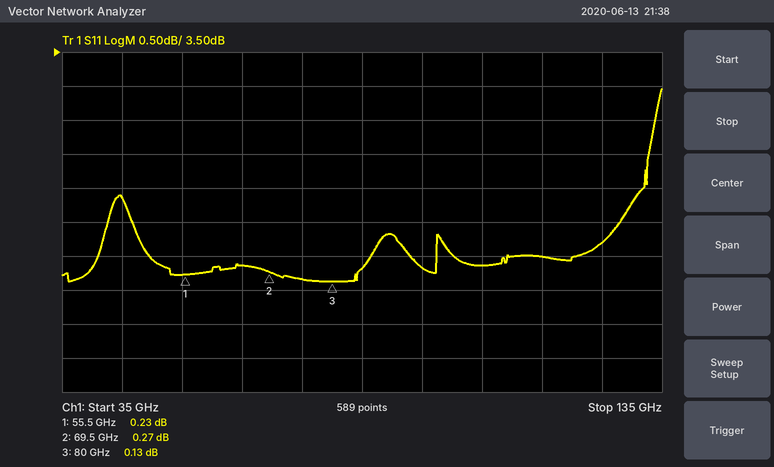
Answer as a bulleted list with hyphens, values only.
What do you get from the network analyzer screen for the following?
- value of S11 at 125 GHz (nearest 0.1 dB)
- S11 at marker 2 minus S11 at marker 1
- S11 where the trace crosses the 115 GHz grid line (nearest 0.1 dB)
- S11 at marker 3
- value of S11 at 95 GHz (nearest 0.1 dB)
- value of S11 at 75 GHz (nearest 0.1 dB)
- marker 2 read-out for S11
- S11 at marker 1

- 0.7 dB
- 0.04 dB
- 0.5 dB
- 0.13 dB
- 0.3 dB
- 0.2 dB
- 0.27 dB
- 0.23 dB
